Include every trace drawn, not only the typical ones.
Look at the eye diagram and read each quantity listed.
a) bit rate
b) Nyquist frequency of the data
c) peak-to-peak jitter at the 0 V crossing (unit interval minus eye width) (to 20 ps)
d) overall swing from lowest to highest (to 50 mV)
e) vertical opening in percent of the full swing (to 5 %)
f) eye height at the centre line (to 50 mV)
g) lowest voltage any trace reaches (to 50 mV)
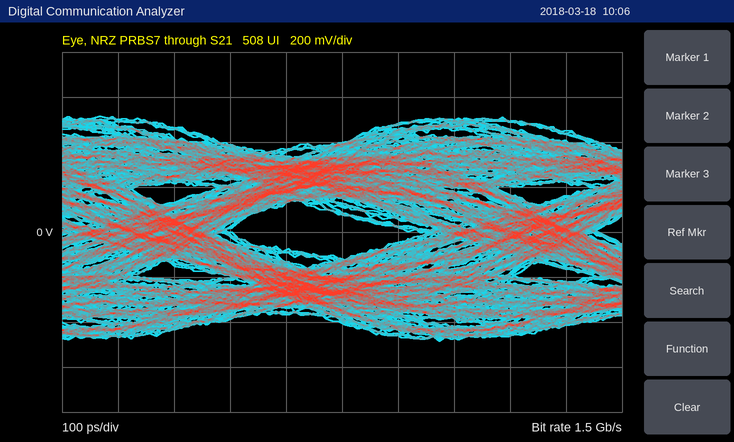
1.5 Gb/s
750 MHz
320 ps
1.00 V
20 %
200 mV
-500 mV
